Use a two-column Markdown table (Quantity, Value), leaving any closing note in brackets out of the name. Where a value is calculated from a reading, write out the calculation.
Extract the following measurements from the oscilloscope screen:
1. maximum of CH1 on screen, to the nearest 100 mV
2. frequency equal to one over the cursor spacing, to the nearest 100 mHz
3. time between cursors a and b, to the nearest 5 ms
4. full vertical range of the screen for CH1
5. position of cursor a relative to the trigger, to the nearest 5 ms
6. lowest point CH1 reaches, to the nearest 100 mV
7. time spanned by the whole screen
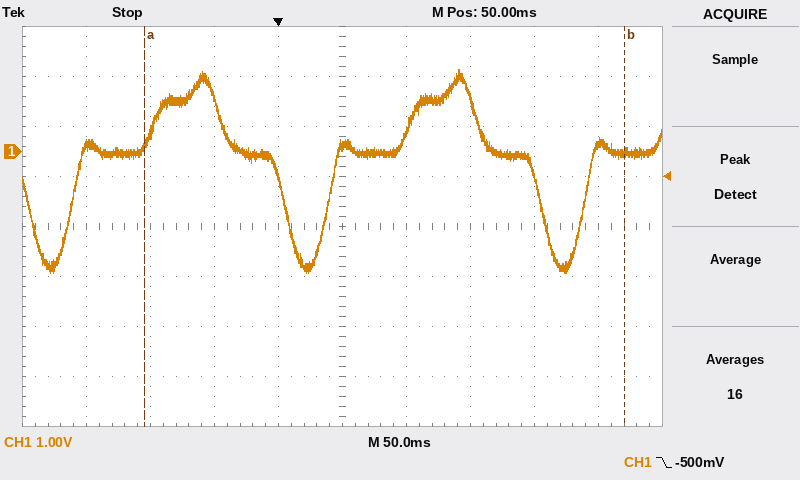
| Quantity | Value |
|---|---|
| maximum of CH1 on screen, to the nearest 100 mV | 1.6 V |
| frequency equal to one over the cursor spacing, to the nearest 100 mHz | 1 / 375 ms ≈ 2.7 Hz |
| time between cursors a and b, to the nearest 5 ms | 375 ms |
| full vertical range of the screen for CH1 | 8 V |
| position of cursor a relative to the trigger, to the nearest 5 ms | -105 ms |
| lowest point CH1 reaches, to the nearest 100 mV | -2.4 V |
| time spanned by the whole screen | 500 ms |
